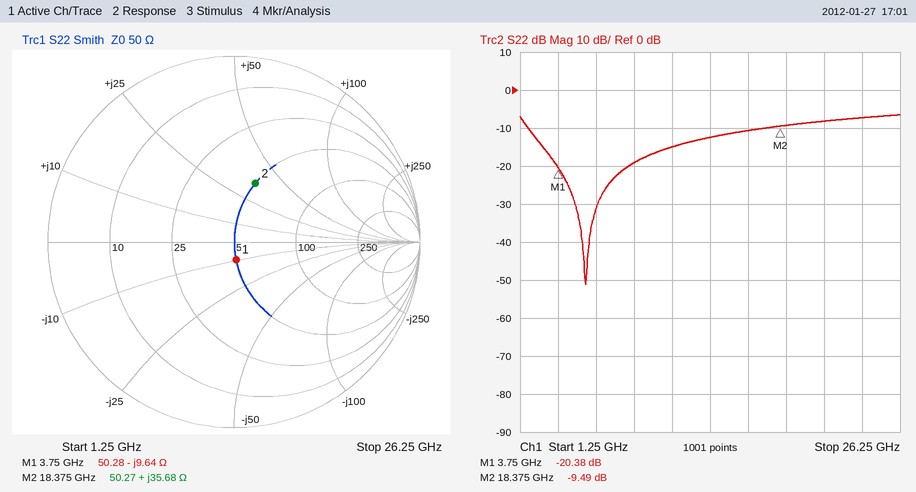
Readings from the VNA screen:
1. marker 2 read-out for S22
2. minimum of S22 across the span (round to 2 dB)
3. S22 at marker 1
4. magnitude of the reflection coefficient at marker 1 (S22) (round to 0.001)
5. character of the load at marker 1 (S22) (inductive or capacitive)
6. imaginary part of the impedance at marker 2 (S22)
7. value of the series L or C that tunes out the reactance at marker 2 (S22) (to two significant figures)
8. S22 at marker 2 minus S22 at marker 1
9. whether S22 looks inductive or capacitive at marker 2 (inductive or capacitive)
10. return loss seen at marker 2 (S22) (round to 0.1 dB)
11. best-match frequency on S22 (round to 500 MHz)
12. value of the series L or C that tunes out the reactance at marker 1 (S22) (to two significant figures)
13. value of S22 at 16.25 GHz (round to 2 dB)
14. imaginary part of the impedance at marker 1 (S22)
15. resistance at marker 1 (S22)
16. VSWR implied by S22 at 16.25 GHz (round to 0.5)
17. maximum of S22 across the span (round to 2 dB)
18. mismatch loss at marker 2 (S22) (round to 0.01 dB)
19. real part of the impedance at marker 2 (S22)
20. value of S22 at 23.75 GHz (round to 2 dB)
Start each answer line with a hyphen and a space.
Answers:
- -9.49 dB
- -52 dB
- -20.38 dB
- 0.096
- capacitive
- +35.68 Ω
- 240 fF
- 10.89 dB
- inductive
- 9.5 dB
- 5.5 GHz
- 410 pH
- -10 dB
- -9.64 Ω
- 50.28 Ω
- 2.0
- -6 dB
- 0.52 dB
- 50.27 Ω
- -8 dB
